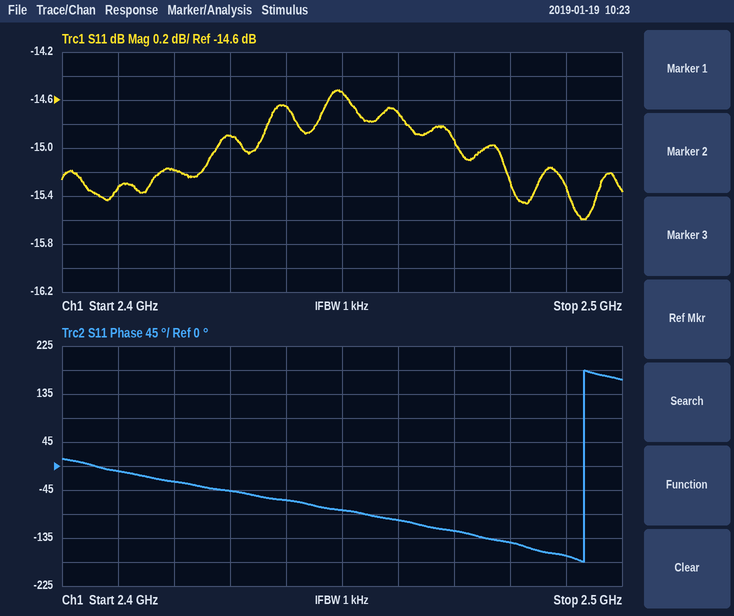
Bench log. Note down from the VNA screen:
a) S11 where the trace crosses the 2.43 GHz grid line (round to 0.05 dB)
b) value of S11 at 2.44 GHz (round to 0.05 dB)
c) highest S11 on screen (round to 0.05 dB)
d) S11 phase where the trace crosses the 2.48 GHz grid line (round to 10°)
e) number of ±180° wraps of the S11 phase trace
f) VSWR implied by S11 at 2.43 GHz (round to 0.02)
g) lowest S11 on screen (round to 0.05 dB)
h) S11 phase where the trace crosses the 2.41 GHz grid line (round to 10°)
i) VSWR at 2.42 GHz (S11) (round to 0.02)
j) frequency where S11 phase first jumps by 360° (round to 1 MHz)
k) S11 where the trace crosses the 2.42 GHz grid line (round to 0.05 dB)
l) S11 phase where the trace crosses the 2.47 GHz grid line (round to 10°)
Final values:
-14.90 dB
-14.65 dB
-14.50 dB
-140°
1
1.44
-15.60 dB
-10°
1.42
2.493 GHz
-15.20 dB
-120°
